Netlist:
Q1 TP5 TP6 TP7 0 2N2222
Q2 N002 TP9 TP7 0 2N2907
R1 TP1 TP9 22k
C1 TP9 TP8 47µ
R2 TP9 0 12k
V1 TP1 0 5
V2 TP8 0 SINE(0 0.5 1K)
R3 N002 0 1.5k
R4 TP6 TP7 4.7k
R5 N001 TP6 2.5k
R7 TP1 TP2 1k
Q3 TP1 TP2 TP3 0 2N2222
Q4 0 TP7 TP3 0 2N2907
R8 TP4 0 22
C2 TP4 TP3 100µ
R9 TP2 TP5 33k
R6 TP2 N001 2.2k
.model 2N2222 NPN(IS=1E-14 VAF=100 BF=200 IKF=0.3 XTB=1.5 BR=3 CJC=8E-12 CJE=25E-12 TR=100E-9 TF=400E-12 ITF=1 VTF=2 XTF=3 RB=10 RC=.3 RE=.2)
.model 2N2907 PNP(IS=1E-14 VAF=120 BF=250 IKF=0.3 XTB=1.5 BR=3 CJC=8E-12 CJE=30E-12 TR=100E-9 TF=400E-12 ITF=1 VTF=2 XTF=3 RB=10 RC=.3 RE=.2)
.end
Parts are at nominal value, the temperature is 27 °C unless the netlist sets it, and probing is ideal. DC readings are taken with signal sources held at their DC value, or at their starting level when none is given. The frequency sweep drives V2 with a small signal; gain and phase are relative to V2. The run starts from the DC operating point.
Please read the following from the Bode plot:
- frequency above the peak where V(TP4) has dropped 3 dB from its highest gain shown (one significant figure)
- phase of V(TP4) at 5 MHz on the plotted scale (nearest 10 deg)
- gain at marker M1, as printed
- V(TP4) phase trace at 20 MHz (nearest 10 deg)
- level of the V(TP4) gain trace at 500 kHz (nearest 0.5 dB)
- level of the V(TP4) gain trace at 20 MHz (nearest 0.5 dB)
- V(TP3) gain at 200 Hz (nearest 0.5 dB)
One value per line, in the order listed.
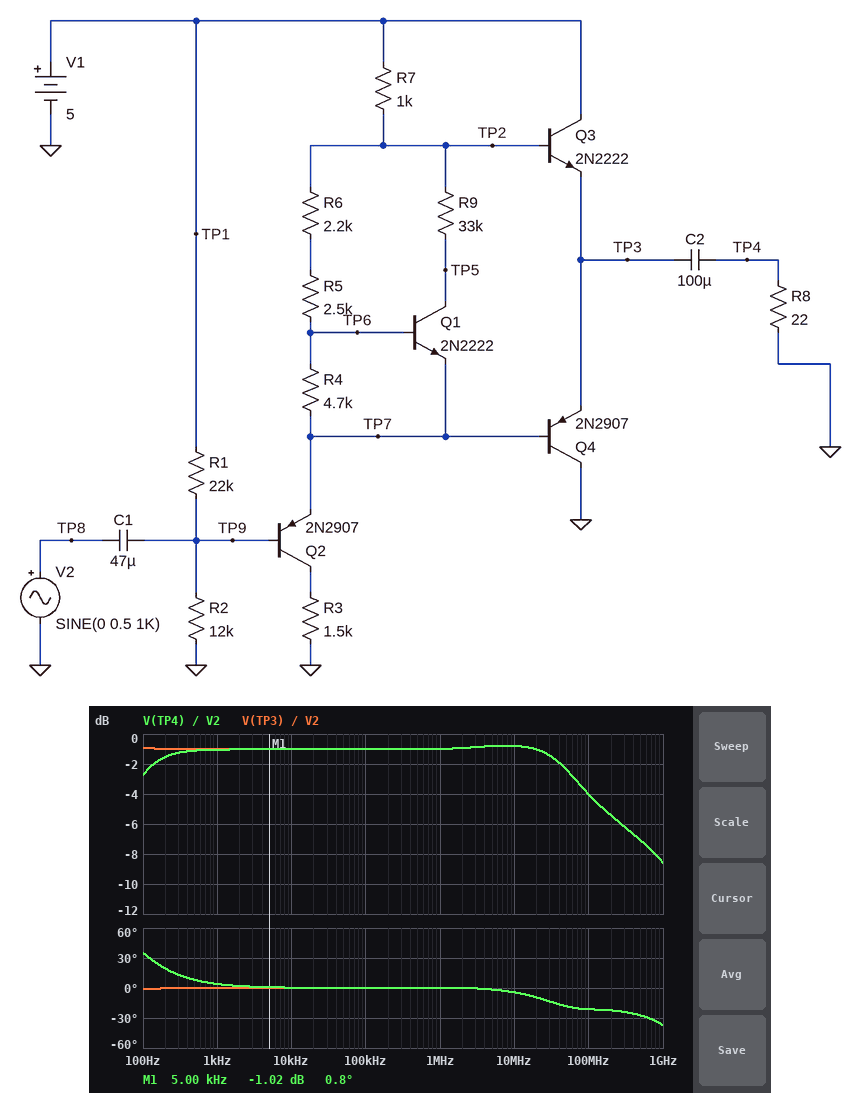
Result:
90 MHz
0 deg
-1.02 dB
-10 deg
-1.0 dB
-1.0 dB
-1.0 dB
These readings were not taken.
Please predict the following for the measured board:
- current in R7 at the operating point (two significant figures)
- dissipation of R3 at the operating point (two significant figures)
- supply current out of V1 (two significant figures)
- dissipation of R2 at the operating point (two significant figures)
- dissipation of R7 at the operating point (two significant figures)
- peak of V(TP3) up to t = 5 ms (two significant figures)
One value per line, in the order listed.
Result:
940 µA
950 µW
100 mA
270 µW
890 µW
3.7 V
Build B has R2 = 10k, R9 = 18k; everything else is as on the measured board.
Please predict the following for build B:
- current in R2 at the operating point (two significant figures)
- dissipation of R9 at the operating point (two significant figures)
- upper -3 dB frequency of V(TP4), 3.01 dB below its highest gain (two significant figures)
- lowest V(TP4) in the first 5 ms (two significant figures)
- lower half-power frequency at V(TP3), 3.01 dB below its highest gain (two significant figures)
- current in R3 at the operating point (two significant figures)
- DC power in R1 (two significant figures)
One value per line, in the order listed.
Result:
160 µA
150 µW
94 MHz
-460 mV
500 mHz
950 µA
530 µW
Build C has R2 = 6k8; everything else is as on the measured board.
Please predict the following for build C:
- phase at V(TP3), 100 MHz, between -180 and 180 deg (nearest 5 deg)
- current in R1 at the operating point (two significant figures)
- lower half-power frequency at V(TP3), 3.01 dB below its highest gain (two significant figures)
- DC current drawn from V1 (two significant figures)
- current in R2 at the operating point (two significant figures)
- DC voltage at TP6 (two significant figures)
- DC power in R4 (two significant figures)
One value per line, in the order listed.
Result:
-25 deg
170 µA
1.8 Hz
160 mA
180 µA
2.5 V
85 µW
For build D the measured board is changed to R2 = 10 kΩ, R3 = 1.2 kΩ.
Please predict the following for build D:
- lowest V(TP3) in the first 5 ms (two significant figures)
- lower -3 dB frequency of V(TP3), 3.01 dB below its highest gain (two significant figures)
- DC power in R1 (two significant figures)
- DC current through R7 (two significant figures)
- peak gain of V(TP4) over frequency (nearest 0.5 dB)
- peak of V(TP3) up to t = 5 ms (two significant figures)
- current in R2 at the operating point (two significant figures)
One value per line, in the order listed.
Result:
2.6 V
500 mHz
530 µW
1.1 mA
-0.5 dB
3.5 V
160 µA
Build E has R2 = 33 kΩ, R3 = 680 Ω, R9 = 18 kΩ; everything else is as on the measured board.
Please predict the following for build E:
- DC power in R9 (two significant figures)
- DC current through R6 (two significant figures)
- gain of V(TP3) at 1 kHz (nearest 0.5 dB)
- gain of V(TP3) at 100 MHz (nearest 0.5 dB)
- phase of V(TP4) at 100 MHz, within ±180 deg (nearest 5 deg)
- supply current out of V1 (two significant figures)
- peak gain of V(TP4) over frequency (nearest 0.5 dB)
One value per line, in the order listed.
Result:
71 µW
130 µA
-21.5 dB
-12.5 dB
40 deg
380 µA
-8.0 dB
